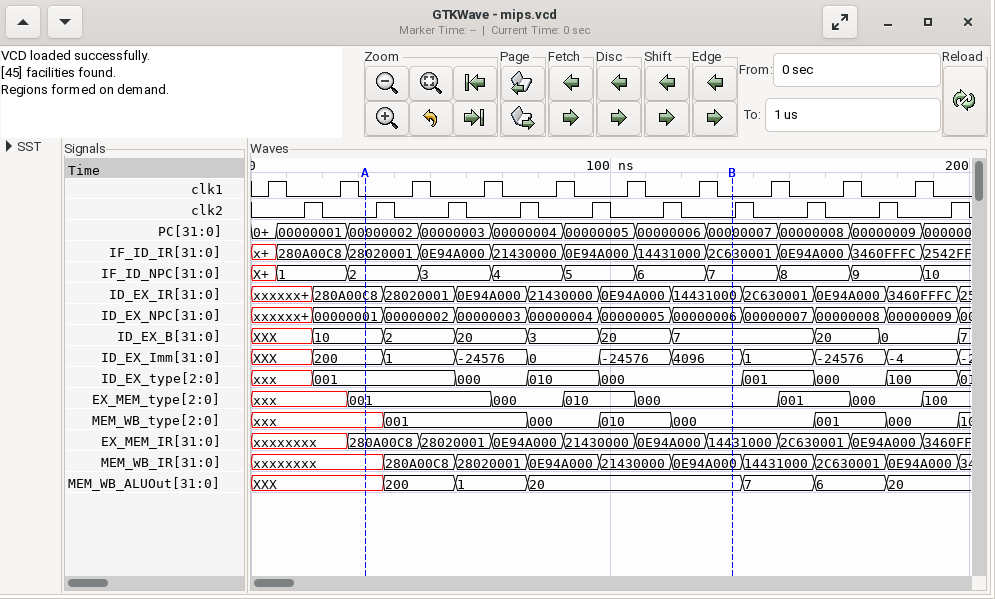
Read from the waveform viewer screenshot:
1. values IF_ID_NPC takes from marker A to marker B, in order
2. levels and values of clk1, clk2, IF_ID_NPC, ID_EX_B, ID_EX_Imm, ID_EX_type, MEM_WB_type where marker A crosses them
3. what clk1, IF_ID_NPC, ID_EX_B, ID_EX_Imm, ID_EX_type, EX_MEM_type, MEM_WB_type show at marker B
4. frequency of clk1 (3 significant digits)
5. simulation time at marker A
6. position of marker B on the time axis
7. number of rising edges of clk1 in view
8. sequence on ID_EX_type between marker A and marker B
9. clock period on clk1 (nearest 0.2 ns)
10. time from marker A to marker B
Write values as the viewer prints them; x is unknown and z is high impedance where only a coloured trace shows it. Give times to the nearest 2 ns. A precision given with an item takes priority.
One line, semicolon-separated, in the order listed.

2, 3, 4, 5, 6, 7; clk1=0, clk2=0, IF_ID_NPC=2, ID_EX_B=10, ID_EX_Imm=200, ID_EX_type=001, MEM_WB_type=xxx; clk1=0, IF_ID_NPC=7, ID_EX_B=7, ID_EX_Imm=4096, ID_EX_type=000, EX_MEM_type=000, MEM_WB_type=000; 50.0 MHz; 32 ns; 134 ns; 10; 001, 000, 010, 000; 20 ns; 102 ns
